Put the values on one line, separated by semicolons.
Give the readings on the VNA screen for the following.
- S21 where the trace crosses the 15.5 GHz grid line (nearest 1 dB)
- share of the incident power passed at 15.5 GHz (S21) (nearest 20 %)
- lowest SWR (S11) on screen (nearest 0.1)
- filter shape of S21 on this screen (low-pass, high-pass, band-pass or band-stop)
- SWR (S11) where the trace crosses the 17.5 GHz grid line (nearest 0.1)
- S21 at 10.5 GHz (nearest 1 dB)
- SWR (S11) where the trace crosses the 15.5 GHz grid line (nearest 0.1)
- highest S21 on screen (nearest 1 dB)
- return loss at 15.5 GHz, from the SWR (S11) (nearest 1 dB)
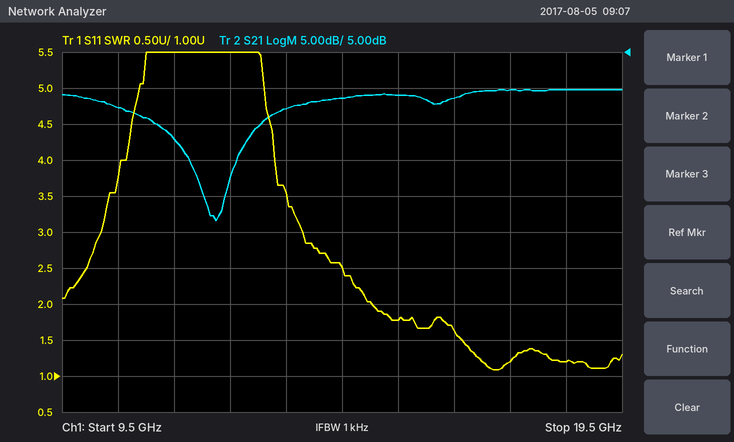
-1 dB; 80 %; 1.1; band-stop; 1.2; -3 dB; 1.8; 0 dB; 11 dB
